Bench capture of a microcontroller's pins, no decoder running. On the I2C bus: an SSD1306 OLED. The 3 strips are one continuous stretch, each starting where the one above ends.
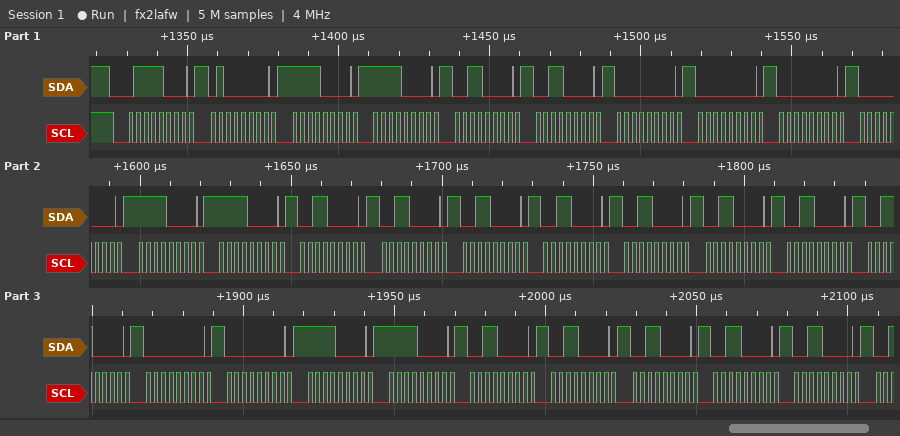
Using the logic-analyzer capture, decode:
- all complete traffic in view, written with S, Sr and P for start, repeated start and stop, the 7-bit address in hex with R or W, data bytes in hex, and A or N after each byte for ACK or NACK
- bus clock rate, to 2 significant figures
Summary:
S 3CW A 40 A F0 A F0 A 30 A 30 A 00 A 00 A 00 A 00 A F0 A F0 A 30 A 30 A 30 A 30 A 30 A 30 A 30 A 30 A 00 A 00 A F0 A F0 A 30 A 30 A 30 A 30 A 30 A
400 kHz
